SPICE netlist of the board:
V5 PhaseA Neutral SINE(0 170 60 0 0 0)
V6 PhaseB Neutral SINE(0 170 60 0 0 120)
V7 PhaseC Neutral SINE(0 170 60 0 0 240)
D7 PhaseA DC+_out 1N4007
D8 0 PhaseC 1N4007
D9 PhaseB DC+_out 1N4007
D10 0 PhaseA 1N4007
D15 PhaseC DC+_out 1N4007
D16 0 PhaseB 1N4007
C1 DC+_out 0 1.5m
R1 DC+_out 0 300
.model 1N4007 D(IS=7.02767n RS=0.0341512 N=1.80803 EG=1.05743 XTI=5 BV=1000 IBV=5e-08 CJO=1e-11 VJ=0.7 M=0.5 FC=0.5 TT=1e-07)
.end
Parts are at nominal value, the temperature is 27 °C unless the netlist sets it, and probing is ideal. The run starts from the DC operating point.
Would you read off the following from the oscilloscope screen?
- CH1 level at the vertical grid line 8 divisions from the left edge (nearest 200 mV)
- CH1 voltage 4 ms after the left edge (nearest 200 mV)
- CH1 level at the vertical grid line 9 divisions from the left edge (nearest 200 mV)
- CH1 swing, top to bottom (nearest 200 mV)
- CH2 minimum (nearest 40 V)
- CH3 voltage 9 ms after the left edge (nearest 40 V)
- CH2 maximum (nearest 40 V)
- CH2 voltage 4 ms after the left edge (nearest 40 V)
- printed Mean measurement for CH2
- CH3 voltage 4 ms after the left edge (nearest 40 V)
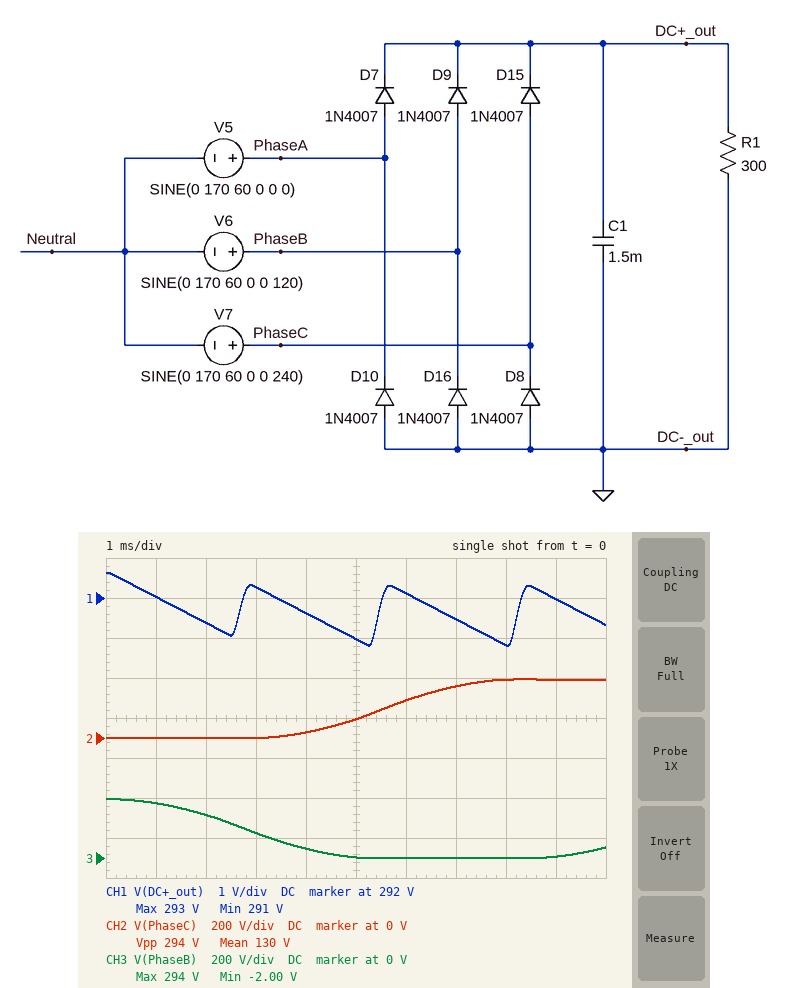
290.8 V
291.6 V
292.0 V
1.8 V
0 V
0 V
280 V
40 V
130 V
40 V
